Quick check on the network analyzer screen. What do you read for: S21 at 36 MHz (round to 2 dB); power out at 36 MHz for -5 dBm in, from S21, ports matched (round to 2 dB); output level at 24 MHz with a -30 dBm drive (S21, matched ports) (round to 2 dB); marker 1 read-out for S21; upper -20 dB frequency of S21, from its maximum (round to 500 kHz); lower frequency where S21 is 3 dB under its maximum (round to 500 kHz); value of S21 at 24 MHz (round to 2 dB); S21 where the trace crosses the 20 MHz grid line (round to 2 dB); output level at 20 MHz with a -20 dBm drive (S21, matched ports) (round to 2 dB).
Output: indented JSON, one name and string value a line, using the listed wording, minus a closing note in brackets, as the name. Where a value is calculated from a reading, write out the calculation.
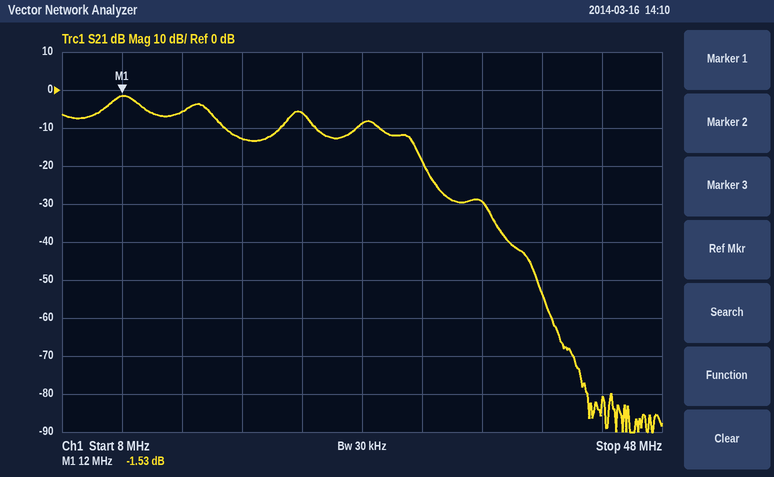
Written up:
{
  "S21 at 36 MHz": "-30 dB",
  "power out at 36 MHz for -5 dBm in, from S21, ports matched": "-5 dBm + (-30 dB) = -34 dBm",
  "output level at 24 MHz with a -30 dBm drive (S21, matched ports)": "-30 dBm + (-6 dB) = -36 dBm",
  "marker 1 read-out for S21": "-1.53 dB",
  "upper -20 dB frequency of S21, from its maximum": "32.5 MHz",
  "lower frequency where S21 is 3 dB under its maximum": "11.0 MHz",
  "value of S21 at 24 MHz": "-6 dB",
  "S21 where the trace crosses the 20 MHz grid line": "-12 dB",
  "output level at 20 MHz with a -20 dBm drive (S21, matched ports)": "-20 dBm + (-12 dB) = -32 dBm"
}
